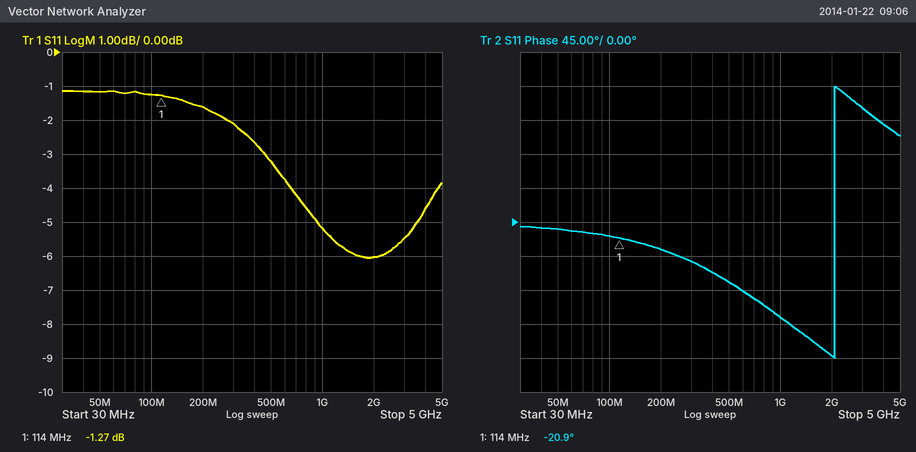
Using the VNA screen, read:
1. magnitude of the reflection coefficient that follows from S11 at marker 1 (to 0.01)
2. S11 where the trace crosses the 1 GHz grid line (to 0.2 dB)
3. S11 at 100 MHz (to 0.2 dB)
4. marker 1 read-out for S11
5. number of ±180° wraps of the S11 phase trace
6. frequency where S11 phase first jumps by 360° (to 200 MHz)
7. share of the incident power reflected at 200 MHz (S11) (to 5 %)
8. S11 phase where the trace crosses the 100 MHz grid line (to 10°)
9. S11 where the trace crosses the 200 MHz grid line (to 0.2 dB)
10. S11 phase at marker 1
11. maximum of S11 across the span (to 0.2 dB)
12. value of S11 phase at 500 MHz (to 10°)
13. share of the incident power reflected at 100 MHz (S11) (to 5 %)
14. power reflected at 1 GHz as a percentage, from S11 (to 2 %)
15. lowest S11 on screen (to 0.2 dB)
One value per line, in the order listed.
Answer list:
0.86
-5.2 dB
-1.2 dB
-1.27 dB
1
2.0 GHz
70 %
-20°
-1.6 dB
-20.9°
-1.2 dB
-80°
75 %
30 %
-6.0 dB
